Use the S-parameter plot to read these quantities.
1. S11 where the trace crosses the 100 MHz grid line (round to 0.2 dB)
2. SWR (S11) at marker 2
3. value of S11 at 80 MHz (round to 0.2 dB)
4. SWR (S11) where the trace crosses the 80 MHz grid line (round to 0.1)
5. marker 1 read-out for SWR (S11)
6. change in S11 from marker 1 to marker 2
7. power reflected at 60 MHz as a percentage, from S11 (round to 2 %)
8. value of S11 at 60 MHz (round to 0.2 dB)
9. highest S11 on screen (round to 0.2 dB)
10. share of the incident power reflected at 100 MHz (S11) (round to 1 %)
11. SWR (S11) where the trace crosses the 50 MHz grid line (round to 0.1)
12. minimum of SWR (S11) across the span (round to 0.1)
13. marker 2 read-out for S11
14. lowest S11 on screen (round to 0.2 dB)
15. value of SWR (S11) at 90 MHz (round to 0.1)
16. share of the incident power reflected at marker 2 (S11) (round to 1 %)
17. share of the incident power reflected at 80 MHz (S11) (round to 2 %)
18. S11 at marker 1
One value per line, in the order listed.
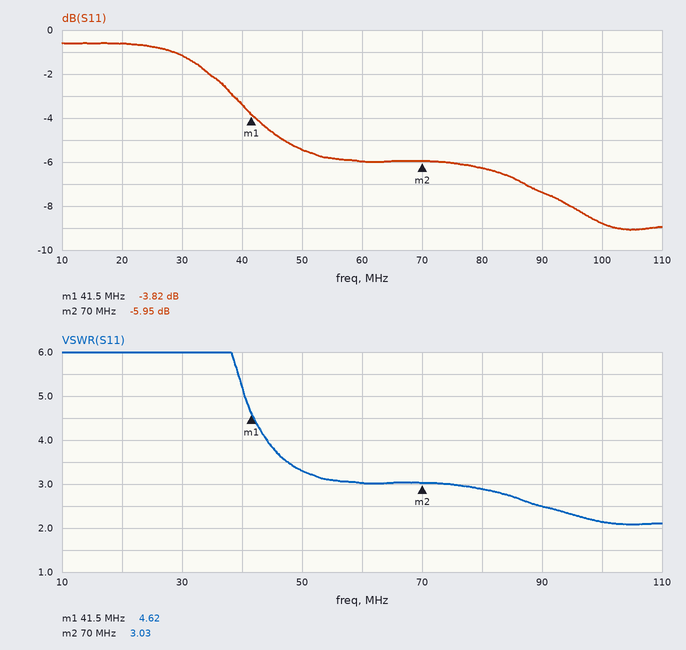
-8.8 dB
3.03
-6.2 dB
2.9
4.62
-2.13 dB
26 %
-6.0 dB
-0.6 dB
13 %
3.3
2.1
-5.95 dB
-9.0 dB
2.5
25 %
24 %
-3.82 dB
